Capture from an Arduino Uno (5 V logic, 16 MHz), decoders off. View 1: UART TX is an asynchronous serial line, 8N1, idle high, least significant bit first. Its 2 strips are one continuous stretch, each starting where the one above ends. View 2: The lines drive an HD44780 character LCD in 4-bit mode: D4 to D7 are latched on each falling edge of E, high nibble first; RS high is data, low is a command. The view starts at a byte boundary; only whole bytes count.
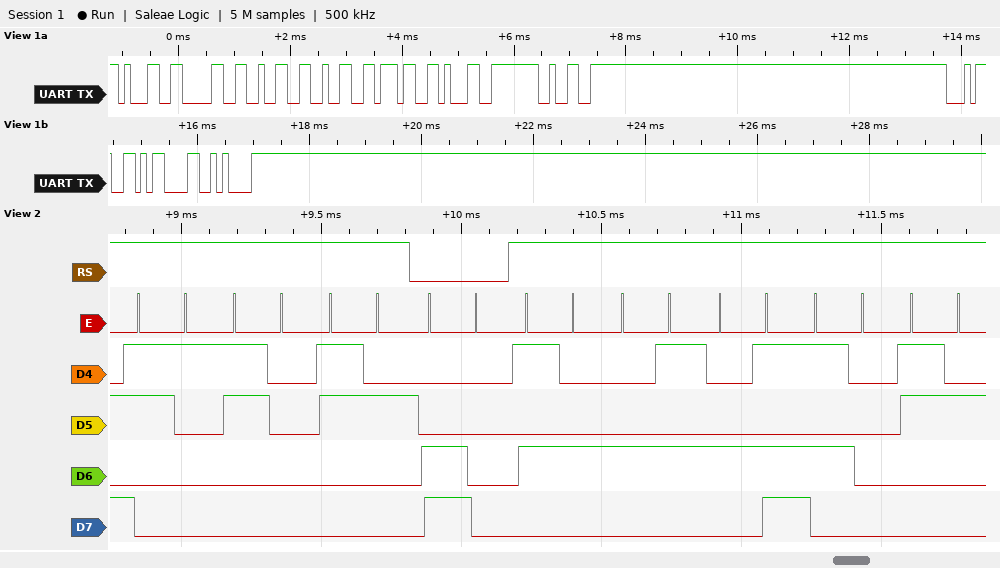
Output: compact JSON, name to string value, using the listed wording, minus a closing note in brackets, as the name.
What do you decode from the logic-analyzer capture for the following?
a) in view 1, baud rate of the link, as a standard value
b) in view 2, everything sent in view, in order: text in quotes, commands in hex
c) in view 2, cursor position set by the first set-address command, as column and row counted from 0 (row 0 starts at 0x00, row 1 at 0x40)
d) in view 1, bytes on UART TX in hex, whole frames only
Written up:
{"in view 1, baud rate of the link, as a standard value": "9600 baud", "in view 2, everything sent in view, in order: text in quotes, commands in hex": "\"102\" 0xC0 \"TEMP2\"", "in view 2, cursor position set by the first set-address command, as column and row counted from 0": "column 0, row 1", "in view 1, bytes on UART TX in hex, whole frames only": "31 30 32 32 37 31 32 34 0D 0A"}
